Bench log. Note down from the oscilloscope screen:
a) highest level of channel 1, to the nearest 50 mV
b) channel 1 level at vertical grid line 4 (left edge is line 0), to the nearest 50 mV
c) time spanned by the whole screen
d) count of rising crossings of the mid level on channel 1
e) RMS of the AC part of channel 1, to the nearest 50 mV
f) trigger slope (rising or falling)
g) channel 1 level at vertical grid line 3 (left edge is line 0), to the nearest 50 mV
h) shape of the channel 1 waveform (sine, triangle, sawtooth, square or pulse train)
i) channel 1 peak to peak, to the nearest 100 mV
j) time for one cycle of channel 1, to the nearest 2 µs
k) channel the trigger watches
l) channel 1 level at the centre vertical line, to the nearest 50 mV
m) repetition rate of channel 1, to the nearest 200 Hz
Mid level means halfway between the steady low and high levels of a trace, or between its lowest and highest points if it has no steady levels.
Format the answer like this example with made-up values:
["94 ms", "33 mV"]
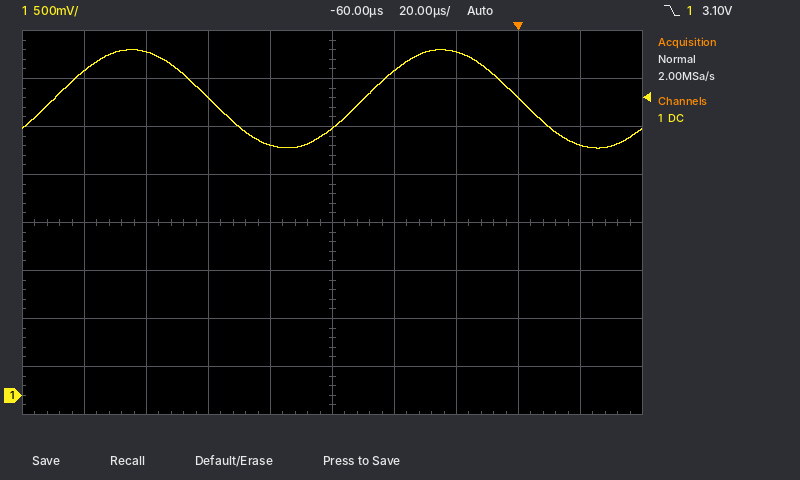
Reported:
["3.60 V", "2.60 V", "200 µs", "2", "350 mV", "falling", "3.10 V", "sine", "1.00 V", "100 µs", "channel 1", "2.80 V", "10.0 kHz"]
